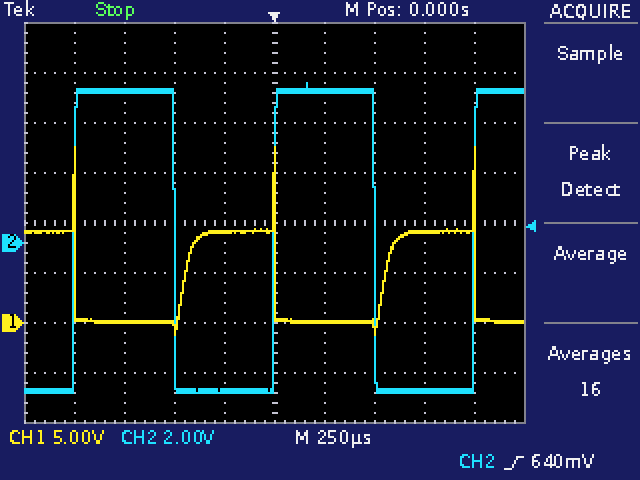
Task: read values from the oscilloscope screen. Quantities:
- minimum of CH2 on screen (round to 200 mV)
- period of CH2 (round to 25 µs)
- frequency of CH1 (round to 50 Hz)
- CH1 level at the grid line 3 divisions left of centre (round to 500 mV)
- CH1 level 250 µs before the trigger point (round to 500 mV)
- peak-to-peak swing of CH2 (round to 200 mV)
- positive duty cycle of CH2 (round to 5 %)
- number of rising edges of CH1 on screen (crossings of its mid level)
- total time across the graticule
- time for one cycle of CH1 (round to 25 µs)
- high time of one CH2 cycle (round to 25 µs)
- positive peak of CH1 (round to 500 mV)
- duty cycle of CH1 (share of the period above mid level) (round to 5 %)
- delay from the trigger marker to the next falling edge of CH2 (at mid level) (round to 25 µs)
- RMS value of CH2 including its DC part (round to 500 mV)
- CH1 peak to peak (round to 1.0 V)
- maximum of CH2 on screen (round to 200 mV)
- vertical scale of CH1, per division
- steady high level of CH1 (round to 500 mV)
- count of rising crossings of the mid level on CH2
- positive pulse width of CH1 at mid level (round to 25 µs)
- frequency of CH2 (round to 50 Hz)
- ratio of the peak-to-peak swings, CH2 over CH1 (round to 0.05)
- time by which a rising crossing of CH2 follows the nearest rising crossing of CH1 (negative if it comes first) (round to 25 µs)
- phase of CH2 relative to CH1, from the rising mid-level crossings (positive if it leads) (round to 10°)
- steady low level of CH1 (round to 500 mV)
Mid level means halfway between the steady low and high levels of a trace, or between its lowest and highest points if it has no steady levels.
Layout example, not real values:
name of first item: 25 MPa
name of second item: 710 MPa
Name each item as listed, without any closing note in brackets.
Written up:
minimum of CH2 on screen: -6.0 V
period of CH2: 1.000 ms
frequency of CH1: 1.00 kHz
CH1 level at the grid line 3 divisions left of centre: 0.0 V
CH1 level 250 µs before the trigger point: 9.0 V
peak-to-peak swing of CH2: 12.4 V
positive duty cycle of CH2: 50 %
number of rising edges of CH1 on screen: 2
total time across the graticule: 2.5 ms
time for one cycle of CH1: 1.000 ms
high time of one CH2 cycle: 500 µs
positive peak of CH1: 17.5 V
duty cycle of CH1 (share of the period above mid level): 45 %
delay from the trigger marker to the next falling edge of CH2 (at mid level): 500 µs
RMS value of CH2 including its DC part: 6.0 V
CH1 peak to peak: 19.0 V
maximum of CH2 on screen: 6.4 V
vertical scale of CH1, per division: 5 V
steady high level of CH1: 9.0 V
count of rising crossings of the mid level on CH2: 3
positive pulse width of CH1 at mid level: 450 µs
frequency of CH2: 1.00 kHz
ratio of the peak-to-peak swings, CH2 over CH1: 0.65
time by which a rising crossing of CH2 follows the nearest rising crossing of CH1 (negative if it comes first): +450 µs
phase of CH2 relative to CH1, from the rising mid-level crossings (positive if it leads): -160°
steady low level of CH1: 0.0 V
